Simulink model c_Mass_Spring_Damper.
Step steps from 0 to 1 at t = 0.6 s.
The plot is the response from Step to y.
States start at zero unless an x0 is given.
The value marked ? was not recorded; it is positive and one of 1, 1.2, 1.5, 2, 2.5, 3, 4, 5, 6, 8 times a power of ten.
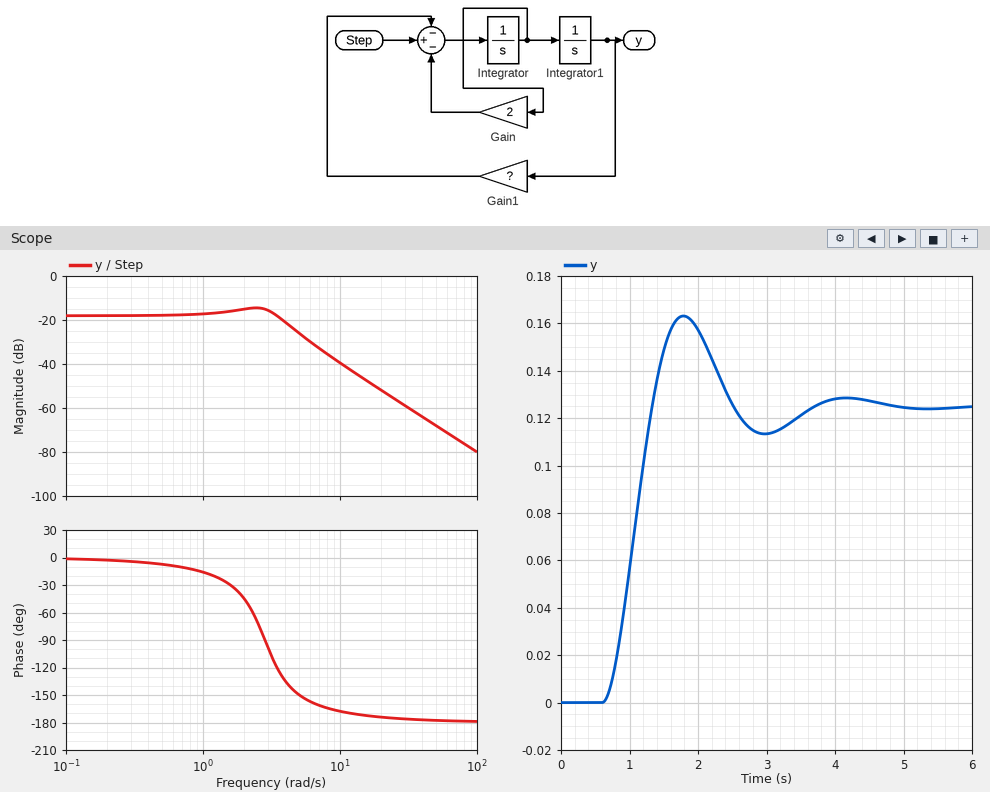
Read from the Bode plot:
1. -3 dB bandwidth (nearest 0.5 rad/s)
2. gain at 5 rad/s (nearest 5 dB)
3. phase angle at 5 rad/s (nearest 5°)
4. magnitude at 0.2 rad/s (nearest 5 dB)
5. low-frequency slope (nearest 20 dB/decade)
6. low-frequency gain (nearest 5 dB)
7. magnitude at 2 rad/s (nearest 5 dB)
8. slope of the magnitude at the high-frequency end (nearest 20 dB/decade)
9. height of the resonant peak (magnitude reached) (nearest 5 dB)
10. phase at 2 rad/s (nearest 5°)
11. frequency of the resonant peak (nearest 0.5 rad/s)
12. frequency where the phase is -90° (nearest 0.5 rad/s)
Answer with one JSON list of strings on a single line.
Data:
["4.0 rad/s", "-25 dB", "-150°", "-20 dB", "0 dB/decade", "-20 dB", "-15 dB", "-40 dB/decade", "-15 dB", "-45°", "2.5 rad/s", "3.0 rad/s"]
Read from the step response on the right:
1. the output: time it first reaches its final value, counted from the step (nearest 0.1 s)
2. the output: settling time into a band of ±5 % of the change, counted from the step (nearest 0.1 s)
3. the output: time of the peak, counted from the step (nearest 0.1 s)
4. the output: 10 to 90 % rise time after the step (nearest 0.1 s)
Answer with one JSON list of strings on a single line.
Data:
["0.7 s", "2.8 s", "1.2 s", "0.5 s"]
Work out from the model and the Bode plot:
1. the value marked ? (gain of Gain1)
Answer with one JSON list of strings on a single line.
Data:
["8"]
